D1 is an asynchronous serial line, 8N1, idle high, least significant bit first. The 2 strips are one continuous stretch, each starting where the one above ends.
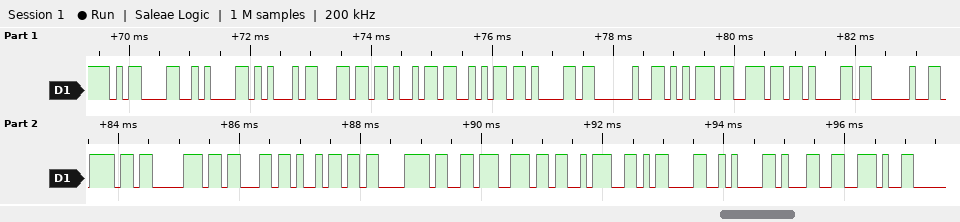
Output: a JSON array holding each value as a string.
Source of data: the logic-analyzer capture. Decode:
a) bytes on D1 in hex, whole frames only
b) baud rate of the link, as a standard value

["0x0D 0x0A 0x45 0x6C 0x69 0x6A 0x61 0x20 0x75 0x6E 0x61 0x20 0x6F 0x70 0x63 0x69 0xC3 0xB3 0x6E 0x3A 0x0D 0x0A 0x31 0x2E", "9600 baud"]
